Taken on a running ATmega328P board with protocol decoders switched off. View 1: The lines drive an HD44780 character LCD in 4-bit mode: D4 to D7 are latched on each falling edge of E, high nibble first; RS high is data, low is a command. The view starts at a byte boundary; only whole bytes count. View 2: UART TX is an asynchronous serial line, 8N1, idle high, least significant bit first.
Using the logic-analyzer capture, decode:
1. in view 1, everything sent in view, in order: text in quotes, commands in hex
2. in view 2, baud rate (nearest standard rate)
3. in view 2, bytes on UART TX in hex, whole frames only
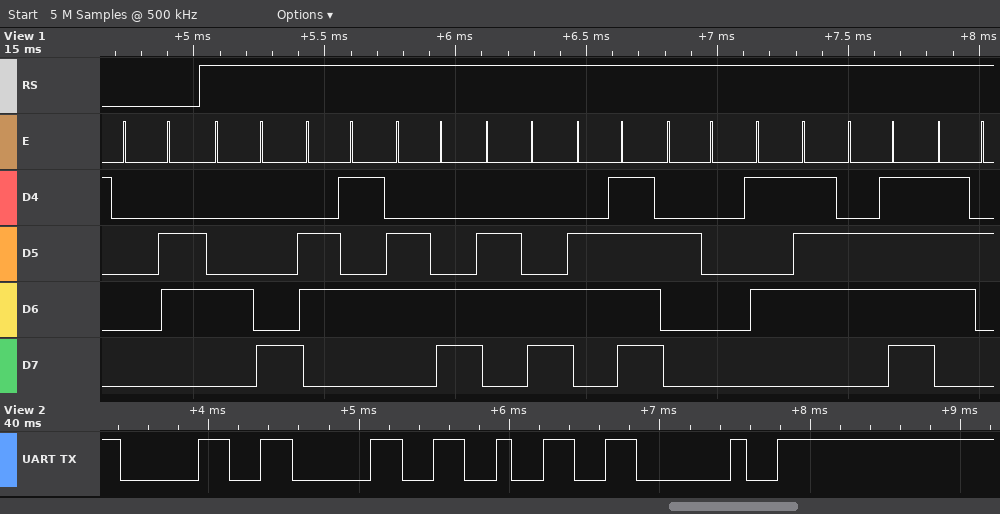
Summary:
0x06 "Hello Wor"
9600 baud
30 30 32 20
